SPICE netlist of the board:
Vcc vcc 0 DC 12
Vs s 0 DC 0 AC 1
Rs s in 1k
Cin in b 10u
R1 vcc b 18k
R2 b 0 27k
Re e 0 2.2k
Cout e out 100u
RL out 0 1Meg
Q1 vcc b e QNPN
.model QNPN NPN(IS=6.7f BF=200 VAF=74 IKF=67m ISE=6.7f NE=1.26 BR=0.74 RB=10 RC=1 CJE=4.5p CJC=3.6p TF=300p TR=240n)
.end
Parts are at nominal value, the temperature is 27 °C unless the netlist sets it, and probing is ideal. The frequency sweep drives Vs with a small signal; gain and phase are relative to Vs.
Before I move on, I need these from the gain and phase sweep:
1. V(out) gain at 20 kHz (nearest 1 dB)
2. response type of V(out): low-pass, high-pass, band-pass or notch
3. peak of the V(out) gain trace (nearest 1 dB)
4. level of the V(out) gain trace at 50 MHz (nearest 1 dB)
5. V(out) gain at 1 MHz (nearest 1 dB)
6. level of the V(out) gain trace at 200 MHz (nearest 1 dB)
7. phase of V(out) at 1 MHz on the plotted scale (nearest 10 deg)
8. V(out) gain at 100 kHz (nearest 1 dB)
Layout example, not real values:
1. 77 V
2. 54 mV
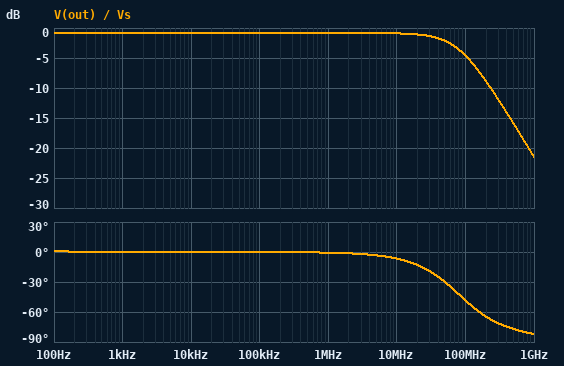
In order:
1. -1 dB
2. low-pass
3. -1 dB
4. -2 dB
5. -1 dB
6. -9 dB
7. 0 deg
8. -1 dB
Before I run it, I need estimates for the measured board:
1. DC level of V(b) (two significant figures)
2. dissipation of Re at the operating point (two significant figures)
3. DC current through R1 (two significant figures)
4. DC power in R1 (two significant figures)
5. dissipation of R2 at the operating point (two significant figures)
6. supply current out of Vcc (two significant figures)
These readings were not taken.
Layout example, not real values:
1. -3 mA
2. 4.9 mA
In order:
1. 6.9 V
2. 18 mW
3. 280 µA
4. 1.4 mW
5. 1.8 mW
6. 3.1 mA
